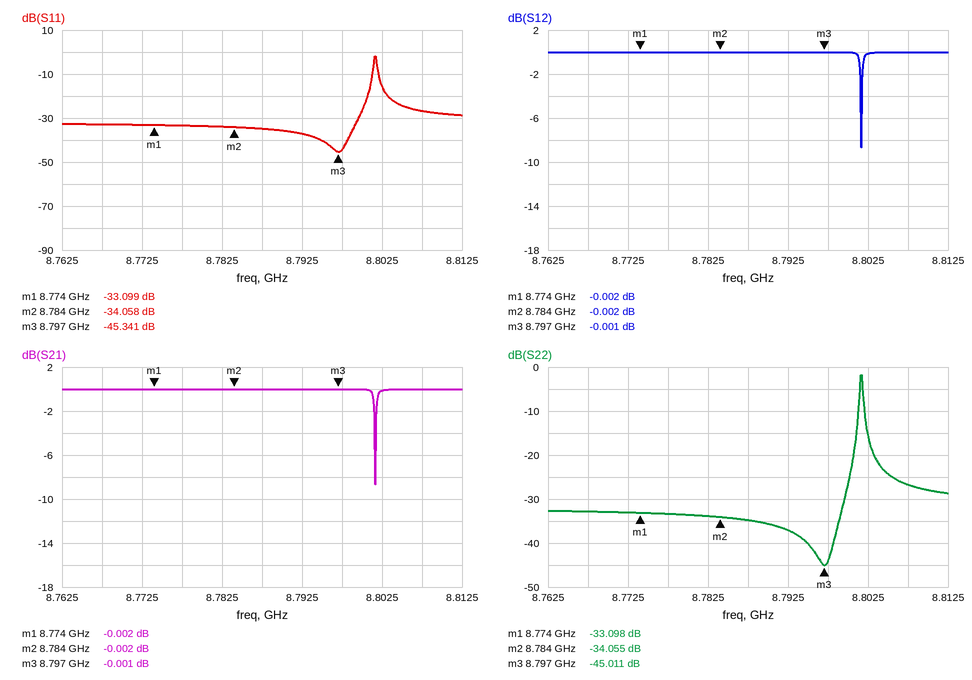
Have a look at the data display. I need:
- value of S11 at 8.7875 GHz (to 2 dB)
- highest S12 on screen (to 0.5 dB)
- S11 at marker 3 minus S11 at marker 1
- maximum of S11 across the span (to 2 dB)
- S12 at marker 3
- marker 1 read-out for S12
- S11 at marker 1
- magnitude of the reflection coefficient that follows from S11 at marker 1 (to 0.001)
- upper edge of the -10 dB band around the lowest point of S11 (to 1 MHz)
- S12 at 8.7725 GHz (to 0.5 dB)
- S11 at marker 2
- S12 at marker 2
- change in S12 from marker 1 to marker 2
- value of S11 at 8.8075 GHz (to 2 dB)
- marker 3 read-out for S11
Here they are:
-34 dB
0.0 dB
-12.242 dB
-2 dB
-0.001 dB
-0.002 dB
-33.099 dB
0.022
8.801 GHz
0.0 dB
-34.058 dB
-0.002 dB
0.000 dB
-26 dB
-45.341 dB
